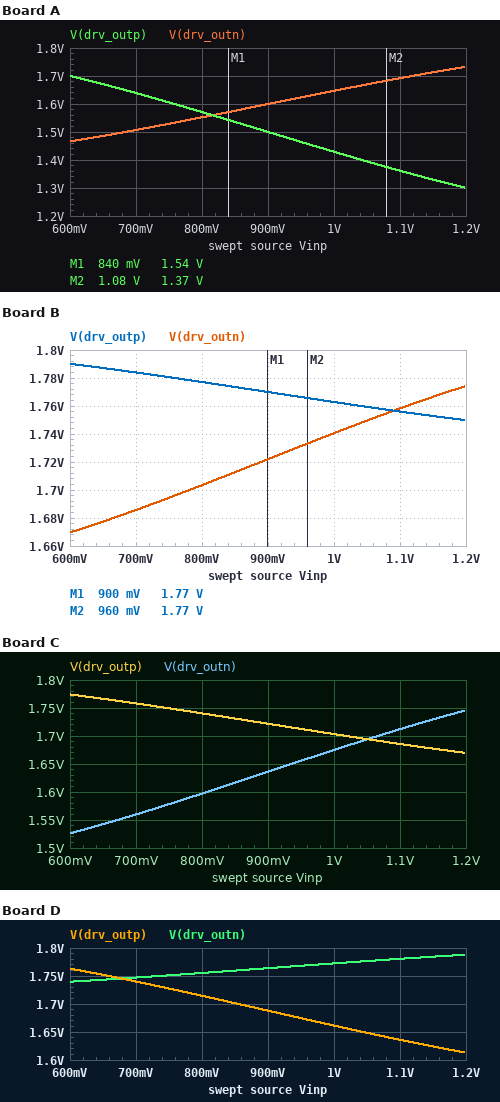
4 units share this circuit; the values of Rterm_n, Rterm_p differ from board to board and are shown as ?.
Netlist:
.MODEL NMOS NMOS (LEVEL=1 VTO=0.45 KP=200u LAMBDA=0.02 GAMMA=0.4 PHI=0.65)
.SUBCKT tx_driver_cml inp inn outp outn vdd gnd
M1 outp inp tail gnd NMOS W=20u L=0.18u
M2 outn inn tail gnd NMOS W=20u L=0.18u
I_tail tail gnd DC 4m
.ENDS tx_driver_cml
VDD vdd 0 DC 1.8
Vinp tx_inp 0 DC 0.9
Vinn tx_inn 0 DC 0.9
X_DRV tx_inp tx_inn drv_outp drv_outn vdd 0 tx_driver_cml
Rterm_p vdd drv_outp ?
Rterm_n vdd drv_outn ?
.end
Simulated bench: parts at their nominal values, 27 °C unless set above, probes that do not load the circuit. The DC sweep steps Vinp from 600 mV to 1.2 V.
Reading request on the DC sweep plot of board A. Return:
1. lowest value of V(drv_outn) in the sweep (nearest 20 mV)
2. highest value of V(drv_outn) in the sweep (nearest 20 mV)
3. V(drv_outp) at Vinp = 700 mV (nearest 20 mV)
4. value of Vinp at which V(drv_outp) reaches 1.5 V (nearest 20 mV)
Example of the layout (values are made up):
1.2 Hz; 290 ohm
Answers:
1.46 V; 1.74 V; 1.64 V; 900 mV
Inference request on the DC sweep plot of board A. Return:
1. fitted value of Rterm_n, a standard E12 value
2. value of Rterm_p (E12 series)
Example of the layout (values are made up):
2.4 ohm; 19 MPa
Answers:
100 Ω; 150 Ω
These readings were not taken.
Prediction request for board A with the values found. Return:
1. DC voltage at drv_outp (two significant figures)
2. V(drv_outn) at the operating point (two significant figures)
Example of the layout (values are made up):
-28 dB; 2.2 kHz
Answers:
1.5 V; 1.6 V
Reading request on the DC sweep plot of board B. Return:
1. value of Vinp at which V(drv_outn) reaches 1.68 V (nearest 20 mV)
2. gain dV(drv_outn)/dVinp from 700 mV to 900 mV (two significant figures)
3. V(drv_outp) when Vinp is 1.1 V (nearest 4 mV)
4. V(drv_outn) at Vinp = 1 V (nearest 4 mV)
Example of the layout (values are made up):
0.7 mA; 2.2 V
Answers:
660 mV; 0.18 V/V; 1.756 V; 1.740 V
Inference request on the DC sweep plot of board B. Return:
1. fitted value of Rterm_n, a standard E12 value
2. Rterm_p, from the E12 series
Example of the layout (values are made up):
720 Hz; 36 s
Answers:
39 Ω; 15 Ω
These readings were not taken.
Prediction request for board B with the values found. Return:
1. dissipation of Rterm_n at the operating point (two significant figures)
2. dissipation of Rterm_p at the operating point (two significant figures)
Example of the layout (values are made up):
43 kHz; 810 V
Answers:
160 µW; 60 µW
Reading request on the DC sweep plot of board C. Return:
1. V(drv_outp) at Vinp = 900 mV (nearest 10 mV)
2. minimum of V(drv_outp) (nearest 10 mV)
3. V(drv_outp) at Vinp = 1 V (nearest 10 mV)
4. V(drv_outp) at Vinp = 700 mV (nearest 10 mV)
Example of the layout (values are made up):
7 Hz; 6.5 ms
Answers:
1.72 V; 1.67 V; 1.70 V; 1.76 V
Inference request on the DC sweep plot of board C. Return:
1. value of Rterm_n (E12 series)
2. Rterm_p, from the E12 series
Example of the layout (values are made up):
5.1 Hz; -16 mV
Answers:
82 Ω; 39 Ω
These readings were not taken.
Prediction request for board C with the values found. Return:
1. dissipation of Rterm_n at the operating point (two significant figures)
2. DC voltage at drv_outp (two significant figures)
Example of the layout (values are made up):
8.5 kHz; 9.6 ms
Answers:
330 µW; 1.7 V
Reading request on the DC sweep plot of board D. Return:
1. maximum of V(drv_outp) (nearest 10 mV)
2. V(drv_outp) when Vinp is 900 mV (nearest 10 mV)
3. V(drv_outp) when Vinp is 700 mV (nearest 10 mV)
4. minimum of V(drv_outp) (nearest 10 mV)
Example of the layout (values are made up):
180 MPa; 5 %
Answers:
1.76 V; 1.69 V; 1.74 V; 1.61 V
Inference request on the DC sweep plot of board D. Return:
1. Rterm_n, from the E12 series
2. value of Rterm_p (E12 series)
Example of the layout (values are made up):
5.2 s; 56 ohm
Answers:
18 Ω; 56 Ω
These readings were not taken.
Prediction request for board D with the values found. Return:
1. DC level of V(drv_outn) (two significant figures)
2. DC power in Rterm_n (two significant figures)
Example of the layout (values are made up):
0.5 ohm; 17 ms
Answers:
1.8 V; 72 µW
